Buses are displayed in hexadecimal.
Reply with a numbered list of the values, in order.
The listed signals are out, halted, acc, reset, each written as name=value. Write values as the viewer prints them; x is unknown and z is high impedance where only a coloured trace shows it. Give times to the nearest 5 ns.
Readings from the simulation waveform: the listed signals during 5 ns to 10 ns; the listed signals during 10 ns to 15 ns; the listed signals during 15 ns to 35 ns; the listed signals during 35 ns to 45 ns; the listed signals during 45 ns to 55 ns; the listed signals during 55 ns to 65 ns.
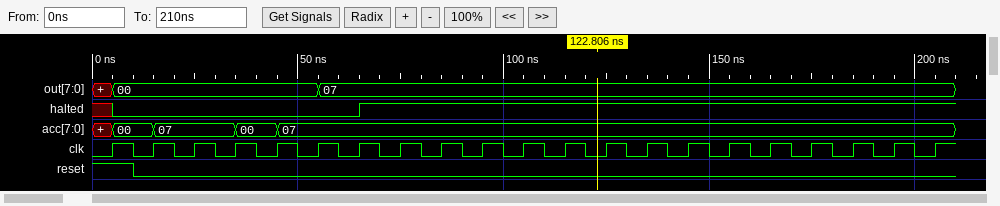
1. out=00, halted=0, acc=00, reset=1
2. out=00, halted=0, acc=00, reset=0
3. out=00, halted=0, acc=07, reset=0
4. out=00, halted=0, acc=00, reset=0
5. out=00, halted=0, acc=07, reset=0
6. out=07, halted=0, acc=07, reset=0
